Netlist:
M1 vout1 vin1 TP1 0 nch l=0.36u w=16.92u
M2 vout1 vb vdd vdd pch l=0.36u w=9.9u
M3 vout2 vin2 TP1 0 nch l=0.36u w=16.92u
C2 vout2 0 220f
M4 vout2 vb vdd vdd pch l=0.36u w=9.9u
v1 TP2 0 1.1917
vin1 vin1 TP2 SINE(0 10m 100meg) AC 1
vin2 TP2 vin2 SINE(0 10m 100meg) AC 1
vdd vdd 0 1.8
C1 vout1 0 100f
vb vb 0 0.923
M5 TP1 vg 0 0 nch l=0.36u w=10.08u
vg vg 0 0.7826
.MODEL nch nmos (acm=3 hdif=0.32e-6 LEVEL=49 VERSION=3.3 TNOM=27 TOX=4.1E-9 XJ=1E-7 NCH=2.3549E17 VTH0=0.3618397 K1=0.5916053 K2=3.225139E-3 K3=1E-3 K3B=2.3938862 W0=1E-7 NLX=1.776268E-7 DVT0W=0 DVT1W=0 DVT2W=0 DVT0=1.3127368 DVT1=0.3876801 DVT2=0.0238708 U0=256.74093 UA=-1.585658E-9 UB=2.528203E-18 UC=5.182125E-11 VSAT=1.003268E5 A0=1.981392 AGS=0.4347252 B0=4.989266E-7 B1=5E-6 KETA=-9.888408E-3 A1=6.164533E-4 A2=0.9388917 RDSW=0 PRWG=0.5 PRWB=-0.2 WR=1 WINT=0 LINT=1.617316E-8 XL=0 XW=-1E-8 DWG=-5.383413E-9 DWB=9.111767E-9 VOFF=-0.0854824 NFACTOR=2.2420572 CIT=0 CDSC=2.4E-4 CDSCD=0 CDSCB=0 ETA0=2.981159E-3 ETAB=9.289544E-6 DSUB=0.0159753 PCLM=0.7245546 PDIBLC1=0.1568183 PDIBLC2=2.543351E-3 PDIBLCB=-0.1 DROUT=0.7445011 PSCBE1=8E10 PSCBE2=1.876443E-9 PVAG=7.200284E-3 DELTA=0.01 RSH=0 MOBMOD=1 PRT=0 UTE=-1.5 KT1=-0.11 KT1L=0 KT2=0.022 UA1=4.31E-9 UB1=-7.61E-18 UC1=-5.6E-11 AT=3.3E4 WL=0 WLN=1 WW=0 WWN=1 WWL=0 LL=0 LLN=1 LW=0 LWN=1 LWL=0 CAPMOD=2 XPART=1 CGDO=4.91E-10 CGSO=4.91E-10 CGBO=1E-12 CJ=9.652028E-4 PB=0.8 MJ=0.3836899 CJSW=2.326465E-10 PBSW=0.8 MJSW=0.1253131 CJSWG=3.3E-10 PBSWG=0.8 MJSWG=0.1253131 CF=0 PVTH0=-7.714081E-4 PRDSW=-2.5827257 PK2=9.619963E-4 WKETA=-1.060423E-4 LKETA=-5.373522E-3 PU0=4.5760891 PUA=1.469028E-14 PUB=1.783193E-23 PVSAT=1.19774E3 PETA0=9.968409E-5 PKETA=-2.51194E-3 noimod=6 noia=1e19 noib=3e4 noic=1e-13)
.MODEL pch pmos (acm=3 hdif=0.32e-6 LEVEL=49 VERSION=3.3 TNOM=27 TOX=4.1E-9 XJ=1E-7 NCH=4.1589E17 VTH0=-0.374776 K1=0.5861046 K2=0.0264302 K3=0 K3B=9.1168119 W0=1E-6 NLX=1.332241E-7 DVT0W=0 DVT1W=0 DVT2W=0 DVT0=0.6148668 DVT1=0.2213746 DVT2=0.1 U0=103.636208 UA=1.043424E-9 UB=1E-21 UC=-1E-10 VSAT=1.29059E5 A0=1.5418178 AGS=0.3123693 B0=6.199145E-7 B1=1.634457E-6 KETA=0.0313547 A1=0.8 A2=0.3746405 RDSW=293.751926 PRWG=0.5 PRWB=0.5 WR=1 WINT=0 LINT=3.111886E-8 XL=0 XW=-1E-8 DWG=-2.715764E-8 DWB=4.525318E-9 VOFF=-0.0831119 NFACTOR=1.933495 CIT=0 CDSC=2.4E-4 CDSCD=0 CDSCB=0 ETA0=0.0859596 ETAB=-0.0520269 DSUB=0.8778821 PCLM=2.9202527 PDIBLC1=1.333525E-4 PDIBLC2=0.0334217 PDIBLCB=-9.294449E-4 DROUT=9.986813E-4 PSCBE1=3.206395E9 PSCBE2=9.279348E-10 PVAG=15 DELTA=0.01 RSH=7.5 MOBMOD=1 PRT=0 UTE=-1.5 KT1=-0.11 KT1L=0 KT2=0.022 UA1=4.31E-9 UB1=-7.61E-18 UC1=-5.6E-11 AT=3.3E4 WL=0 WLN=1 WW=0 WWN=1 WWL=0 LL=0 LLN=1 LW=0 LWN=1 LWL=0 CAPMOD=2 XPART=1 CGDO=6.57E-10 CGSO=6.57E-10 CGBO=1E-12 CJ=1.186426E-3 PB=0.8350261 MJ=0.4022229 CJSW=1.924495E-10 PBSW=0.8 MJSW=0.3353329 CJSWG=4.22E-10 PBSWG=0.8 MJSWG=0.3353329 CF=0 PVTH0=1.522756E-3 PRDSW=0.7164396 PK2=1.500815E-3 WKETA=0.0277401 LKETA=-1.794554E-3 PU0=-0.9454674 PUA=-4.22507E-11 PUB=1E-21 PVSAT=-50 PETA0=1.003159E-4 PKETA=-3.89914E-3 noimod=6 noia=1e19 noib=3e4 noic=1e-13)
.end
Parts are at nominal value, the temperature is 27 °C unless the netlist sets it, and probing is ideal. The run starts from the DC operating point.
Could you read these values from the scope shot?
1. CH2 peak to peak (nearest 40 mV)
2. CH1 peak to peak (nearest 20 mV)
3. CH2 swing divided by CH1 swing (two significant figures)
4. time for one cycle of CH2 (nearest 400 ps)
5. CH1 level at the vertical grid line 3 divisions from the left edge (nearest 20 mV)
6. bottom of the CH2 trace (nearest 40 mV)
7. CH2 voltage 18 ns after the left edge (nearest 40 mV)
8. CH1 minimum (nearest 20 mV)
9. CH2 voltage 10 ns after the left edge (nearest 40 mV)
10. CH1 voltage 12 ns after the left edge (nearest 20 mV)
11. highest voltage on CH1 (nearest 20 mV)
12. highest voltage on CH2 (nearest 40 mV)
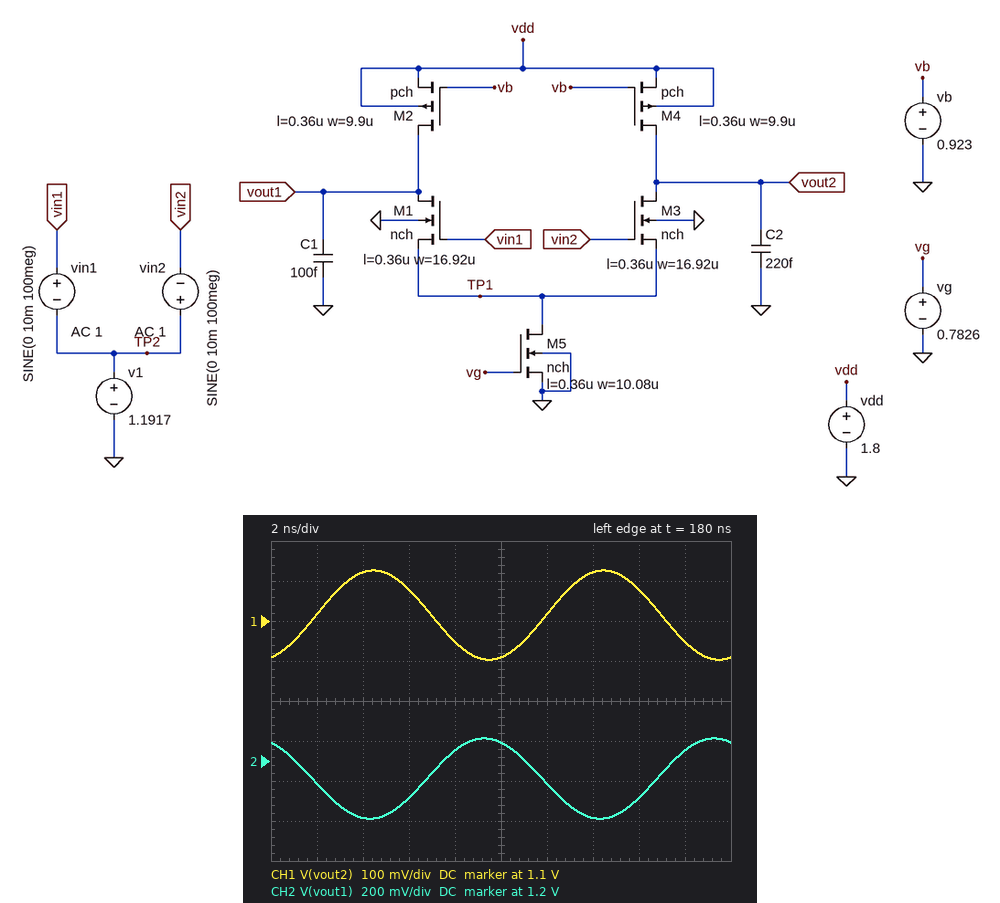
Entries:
400 mV
220 mV
1.8
10.0 ns
1.18 V
920 mV
1.24 V
1.00 V
1.28 V
1.12 V
1.22 V
1.32 V
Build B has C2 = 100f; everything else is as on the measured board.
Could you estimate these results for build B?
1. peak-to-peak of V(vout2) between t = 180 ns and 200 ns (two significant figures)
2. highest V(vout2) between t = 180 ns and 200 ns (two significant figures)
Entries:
390 mV
1.3 V
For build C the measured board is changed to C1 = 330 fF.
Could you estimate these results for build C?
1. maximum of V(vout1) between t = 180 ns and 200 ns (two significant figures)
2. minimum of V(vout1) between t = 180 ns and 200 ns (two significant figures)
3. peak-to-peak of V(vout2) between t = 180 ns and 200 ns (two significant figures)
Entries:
1.2 V
1.0 V
230 mV
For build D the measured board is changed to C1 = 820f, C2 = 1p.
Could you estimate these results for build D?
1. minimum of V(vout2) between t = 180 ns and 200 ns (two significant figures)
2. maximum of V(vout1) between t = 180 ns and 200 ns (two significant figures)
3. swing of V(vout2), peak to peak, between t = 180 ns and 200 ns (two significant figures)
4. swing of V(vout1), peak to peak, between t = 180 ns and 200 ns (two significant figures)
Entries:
1.1 V
1.2 V
60 mV
73 mV
